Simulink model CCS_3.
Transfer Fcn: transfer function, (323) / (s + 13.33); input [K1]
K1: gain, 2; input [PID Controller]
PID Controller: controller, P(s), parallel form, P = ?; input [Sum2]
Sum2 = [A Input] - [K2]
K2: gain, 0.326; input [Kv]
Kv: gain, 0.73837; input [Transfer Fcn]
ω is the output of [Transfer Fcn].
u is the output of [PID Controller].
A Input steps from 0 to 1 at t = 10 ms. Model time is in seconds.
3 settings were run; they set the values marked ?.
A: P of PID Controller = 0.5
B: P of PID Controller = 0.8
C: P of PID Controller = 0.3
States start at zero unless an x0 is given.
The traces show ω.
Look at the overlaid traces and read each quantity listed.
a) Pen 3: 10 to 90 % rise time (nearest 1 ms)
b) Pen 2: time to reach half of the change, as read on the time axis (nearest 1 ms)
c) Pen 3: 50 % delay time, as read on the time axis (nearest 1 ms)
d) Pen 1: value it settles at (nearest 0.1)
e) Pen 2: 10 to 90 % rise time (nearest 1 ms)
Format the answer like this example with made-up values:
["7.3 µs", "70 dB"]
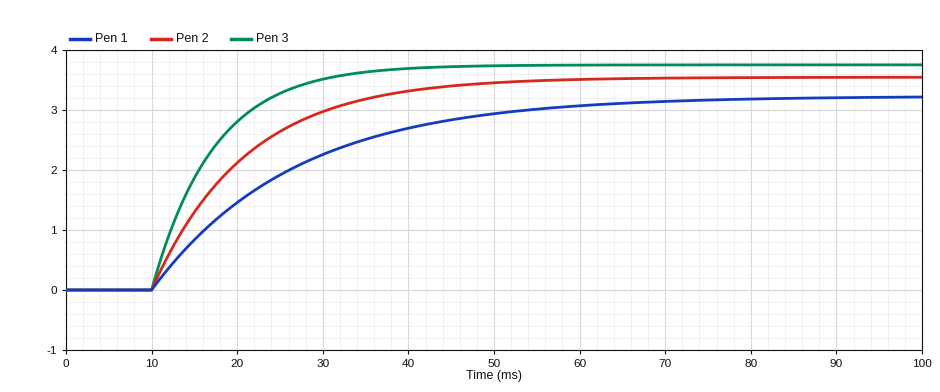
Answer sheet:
["16 ms", "18 ms", "15 ms", "3.2", "24 ms"]
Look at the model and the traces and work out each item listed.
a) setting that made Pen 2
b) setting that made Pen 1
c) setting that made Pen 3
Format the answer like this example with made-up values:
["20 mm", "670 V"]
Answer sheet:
["A", "C", "B"]
